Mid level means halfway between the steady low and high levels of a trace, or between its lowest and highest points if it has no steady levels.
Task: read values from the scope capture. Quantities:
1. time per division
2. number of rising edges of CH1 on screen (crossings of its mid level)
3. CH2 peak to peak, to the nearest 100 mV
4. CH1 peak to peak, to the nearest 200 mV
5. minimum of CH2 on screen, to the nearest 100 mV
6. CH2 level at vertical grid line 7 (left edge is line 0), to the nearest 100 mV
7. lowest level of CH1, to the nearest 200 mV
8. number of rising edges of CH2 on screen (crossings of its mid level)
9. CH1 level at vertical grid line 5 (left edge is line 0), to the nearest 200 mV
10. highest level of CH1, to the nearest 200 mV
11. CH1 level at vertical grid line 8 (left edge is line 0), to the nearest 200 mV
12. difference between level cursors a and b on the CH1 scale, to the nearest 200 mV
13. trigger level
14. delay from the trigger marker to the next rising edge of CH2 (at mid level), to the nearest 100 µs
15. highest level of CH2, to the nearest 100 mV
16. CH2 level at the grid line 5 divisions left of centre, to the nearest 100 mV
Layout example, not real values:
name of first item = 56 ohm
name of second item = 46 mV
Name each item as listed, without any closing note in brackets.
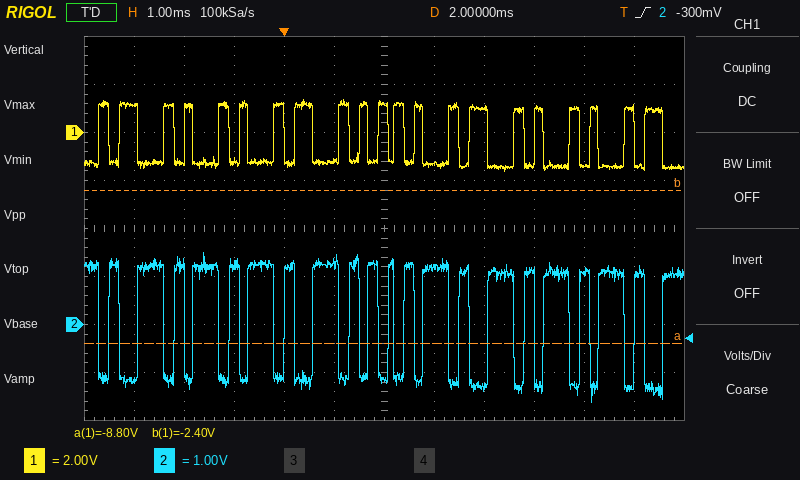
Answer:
time per division = 1 ms
number of rising edges of CH1 on screen = 21
CH2 peak to peak, to the nearest 100 mV = 3.1 V
CH1 peak to peak, to the nearest 200 mV = 3.0 V
minimum of CH2 on screen, to the nearest 100 mV = -1.6 V
CH2 level at vertical grid line 7 (left edge is line 0), to the nearest 100 mV = 1.2 V
lowest level of CH1, to the nearest 200 mV = -1.6 V
number of rising edges of CH2 on screen = 21
CH1 level at vertical grid line 5 (left edge is line 0), to the nearest 200 mV = -1.2 V
highest level of CH1, to the nearest 200 mV = 1.4 V
CH1 level at vertical grid line 8 (left edge is line 0), to the nearest 200 mV = 1.0 V
difference between level cursors a and b on the CH1 scale, to the nearest 200 mV = 6.4 V
trigger level = -300 mV
delay from the trigger marker to the next rising edge of CH2 (at mid level), to the nearest 100 µs = 600 µs
highest level of CH2, to the nearest 100 mV = 1.5 V
CH2 level at the grid line 5 divisions left of centre, to the nearest 100 mV = -1.2 V
